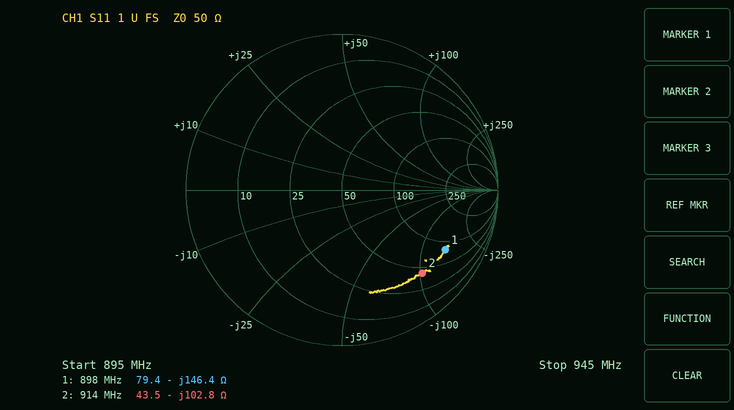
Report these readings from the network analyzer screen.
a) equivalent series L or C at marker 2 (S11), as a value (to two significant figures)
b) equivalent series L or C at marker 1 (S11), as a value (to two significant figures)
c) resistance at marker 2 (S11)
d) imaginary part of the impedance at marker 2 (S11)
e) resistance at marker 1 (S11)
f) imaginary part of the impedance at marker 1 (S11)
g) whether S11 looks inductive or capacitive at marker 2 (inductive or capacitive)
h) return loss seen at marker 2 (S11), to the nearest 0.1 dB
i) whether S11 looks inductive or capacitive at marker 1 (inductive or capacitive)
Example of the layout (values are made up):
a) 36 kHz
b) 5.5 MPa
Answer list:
a) 1.7 pF
b) 1.2 pF
c) 43.5 Ω
d) -102.8 Ω
e) 79.4 Ω
f) -146.4 Ω
g) capacitive
h) 2.6 dB
i) capacitive
